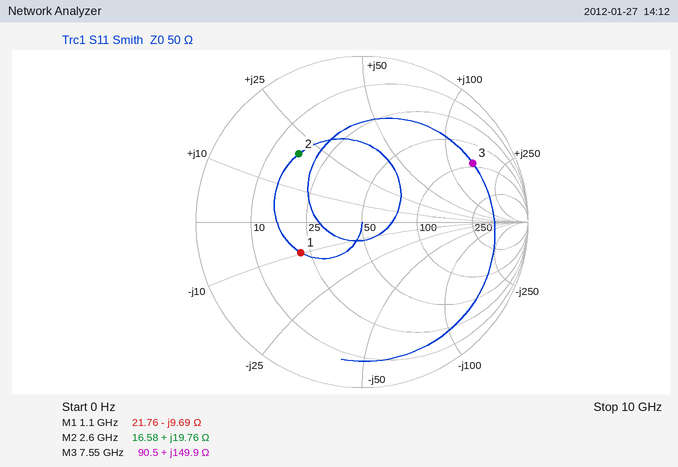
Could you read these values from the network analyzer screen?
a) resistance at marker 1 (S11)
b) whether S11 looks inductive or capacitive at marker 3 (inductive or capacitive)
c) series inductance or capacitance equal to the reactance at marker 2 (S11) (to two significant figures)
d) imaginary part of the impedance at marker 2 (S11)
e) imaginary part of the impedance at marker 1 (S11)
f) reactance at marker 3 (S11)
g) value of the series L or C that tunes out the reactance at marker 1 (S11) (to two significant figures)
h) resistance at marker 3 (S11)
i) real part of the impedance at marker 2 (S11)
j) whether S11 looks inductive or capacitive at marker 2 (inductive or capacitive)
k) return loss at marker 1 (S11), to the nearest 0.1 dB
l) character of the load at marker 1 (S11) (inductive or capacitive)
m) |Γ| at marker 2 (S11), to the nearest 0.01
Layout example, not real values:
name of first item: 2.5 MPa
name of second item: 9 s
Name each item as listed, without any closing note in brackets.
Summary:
resistance at marker 1: 21.76 Ω
whether S11 looks inductive or capacitive at marker 3: inductive
series inductance or capacitance equal to the reactance at marker 2 (S11): 1.2 nH
imaginary part of the impedance at marker 2: +19.76 Ω
imaginary part of the impedance at marker 1: -9.69 Ω
reactance at marker 3: +149.9 Ω
value of the series L or C that tunes out the reactance at marker 1 (S11): 1.4 nH
resistance at marker 3: 90.5 Ω
real part of the impedance at marker 2: 16.58 Ω
whether S11 looks inductive or capacitive at marker 2: inductive
return loss at marker 1 (S11), to the nearest 0.1 dB: 7.7 dB
character of the load at marker 1 (S11): capacitive
|Γ| at marker 2 (S11), to the nearest 0.01: 0.56
